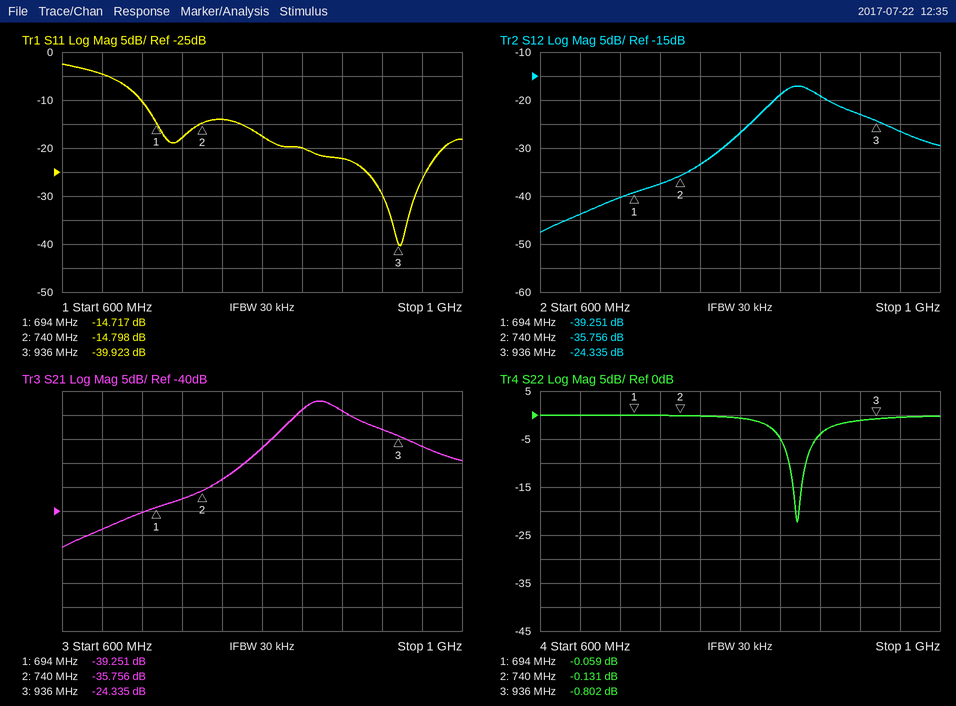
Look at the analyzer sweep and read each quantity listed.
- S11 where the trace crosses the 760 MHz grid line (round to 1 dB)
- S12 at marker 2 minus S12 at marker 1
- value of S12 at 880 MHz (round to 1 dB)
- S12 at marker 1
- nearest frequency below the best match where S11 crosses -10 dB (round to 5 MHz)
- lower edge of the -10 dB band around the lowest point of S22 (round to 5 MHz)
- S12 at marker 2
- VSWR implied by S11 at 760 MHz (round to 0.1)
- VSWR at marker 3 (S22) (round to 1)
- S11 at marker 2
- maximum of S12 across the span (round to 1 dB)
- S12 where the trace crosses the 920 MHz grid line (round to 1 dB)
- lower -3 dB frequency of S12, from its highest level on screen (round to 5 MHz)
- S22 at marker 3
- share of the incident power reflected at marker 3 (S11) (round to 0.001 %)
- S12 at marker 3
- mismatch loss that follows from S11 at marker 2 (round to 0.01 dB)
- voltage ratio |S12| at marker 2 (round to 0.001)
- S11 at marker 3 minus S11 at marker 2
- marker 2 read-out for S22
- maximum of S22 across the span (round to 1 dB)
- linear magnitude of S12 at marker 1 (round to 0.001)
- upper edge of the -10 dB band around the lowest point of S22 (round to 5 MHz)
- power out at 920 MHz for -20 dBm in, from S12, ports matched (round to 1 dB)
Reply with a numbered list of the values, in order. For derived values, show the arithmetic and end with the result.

1. -14 dB
2. -35.756 − (-39.251) = 3.495 dB
3. -19 dB
4. -39.251 dB
5. 680 MHz
6. 850 MHz
7. -35.756 dB
8. |Γ| = 10^(-14/20) = 0.1995; VSWR = (1 + 0.1995)/(1 − 0.1995) ≈ 1.5
9. (1 + 0.9118)/(1 − 0.9118) ≈ 22
10. -14.798 dB
11. -17 dB
12. -23 dB
13. 835 MHz
14. -0.802 dB
15. 10^(-39.923/10) ≈ 0.010 %
16. -24.335 dB
17. −10 log10(1 − 10^(-14.798/10)) ≈ 0.15 dB
18. 10^(-35.756/20) ≈ 0.016
19. -39.923 − (-14.798) = -25.125 dB
20. -0.131 dB
21. 0 dB
22. 10^(-39.251/20) ≈ 0.011
23. 865 MHz
24. -20 dBm + (-23 dB) = -43 dBm
